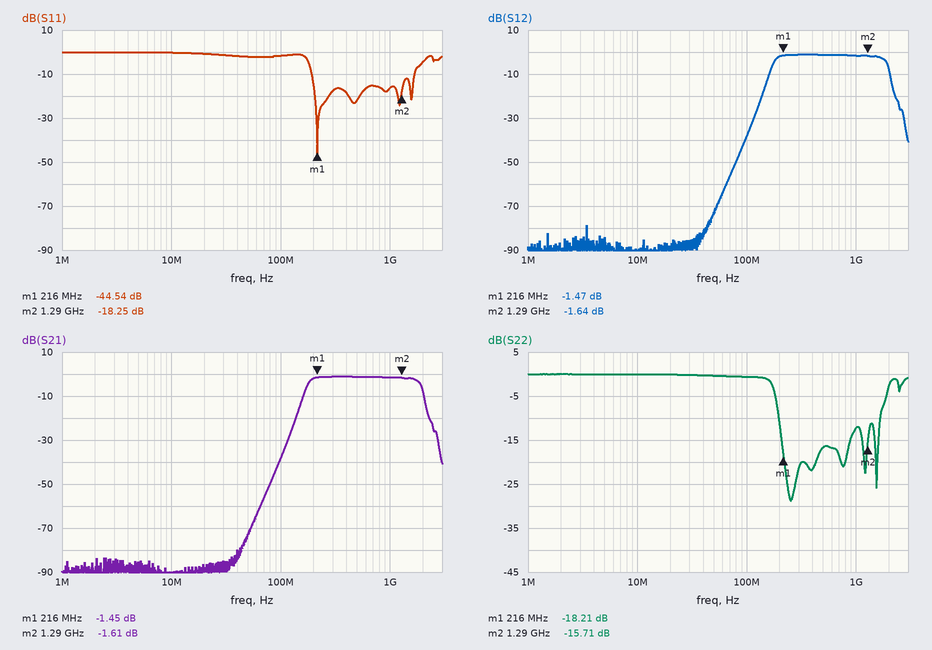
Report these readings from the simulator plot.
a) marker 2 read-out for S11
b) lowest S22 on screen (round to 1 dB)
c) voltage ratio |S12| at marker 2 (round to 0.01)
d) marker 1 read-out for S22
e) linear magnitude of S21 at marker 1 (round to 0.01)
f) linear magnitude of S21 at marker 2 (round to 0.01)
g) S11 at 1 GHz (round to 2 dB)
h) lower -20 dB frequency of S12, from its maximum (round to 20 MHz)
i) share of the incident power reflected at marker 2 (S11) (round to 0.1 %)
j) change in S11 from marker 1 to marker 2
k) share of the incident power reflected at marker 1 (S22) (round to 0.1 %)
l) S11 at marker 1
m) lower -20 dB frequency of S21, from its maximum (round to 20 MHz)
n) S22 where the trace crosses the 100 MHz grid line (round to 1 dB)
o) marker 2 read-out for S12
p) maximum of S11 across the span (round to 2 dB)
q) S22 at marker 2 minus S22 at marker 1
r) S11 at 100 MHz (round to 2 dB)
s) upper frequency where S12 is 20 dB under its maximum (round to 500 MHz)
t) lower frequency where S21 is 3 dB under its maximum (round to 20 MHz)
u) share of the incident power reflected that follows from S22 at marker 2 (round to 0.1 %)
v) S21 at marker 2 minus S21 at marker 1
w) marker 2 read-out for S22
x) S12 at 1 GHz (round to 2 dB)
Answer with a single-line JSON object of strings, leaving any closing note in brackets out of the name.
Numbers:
{"marker 2 read-out for S11": "-18.25 dB", "lowest S22 on screen": "-29 dB", "voltage ratio |S12| at marker 2": "0.83", "marker 1 read-out for S22": "-18.21 dB", "linear magnitude of S21 at marker 1": "0.85", "linear magnitude of S21 at marker 2": "0.83", "S11 at 1 GHz": "-16 dB", "lower -20 dB frequency of S12, from its maximum": "140 MHz", "share of the incident power reflected at marker 2 (S11)": "1.5 %", "change in S11 from marker 1 to marker 2": "26.29 dB", "share of the incident power reflected at marker 1 (S22)": "1.5 %", "S11 at marker 1": "-44.54 dB", "lower -20 dB frequency of S21, from its maximum": "140 MHz", "S22 where the trace crosses the 100 MHz grid line": "-1 dB", "marker 2 read-out for S12": "-1.64 dB", "maximum of S11 across the span": "0 dB", "S22 at marker 2 minus S22 at marker 1": "2.50 dB", "S11 at 100 MHz": "-2 dB", "upper frequency where S12 is 20 dB under its maximum": "2.5 GHz", "lower frequency where S21 is 3 dB under its maximum": "180 MHz", "share of the incident power reflected that follows from S22 at marker 2": "2.7 %", "S21 at marker 2 minus S21 at marker 1": "-0.16 dB", "marker 2 read-out for S22": "-15.71 dB", "S12 at 1 GHz": "-2 dB"}
